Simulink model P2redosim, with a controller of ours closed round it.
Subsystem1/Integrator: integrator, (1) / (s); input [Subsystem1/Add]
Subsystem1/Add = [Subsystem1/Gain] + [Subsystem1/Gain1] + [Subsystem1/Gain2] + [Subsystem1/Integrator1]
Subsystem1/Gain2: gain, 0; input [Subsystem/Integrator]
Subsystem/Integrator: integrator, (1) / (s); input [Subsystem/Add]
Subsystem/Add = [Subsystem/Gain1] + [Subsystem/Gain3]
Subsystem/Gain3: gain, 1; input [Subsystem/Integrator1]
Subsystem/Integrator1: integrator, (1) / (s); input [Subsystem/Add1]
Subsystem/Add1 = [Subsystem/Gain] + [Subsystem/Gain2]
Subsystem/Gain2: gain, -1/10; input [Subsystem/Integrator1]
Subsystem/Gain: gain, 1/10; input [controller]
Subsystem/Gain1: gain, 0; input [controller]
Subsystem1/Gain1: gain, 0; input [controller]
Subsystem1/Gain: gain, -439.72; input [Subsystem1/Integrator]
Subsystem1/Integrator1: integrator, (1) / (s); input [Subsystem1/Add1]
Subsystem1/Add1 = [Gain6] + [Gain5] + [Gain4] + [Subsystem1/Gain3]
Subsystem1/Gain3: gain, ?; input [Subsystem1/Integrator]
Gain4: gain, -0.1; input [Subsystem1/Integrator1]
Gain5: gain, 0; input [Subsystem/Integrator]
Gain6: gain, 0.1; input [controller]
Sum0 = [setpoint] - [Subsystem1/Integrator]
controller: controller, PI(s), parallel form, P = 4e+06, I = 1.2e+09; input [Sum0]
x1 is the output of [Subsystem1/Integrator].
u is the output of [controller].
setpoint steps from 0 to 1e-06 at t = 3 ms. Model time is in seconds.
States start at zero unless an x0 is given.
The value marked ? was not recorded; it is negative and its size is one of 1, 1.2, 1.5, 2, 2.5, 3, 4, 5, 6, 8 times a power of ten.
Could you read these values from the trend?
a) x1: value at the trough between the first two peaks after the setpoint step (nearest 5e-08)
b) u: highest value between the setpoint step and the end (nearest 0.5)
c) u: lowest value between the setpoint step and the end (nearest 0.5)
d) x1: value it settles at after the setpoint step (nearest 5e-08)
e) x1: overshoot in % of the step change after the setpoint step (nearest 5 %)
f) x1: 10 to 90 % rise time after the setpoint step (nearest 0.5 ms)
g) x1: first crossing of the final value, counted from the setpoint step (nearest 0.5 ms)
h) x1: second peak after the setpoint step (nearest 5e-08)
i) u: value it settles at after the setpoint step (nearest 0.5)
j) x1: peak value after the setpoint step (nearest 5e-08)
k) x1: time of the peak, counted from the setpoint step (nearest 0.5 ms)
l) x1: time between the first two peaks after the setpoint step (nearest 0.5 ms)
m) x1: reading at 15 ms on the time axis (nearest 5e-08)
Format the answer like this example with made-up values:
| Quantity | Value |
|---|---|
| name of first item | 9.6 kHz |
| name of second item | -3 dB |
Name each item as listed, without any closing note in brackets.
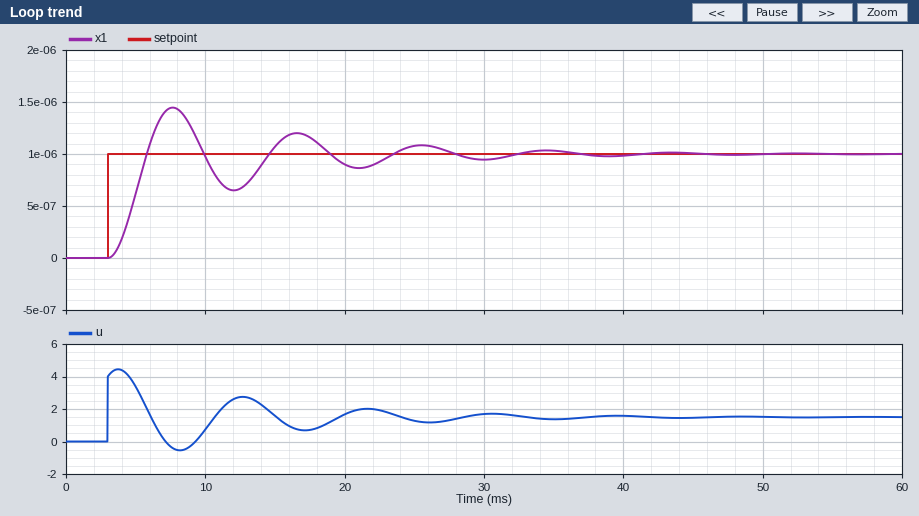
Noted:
| Quantity | Value |
|---|---|
| x1: value at the trough between the first two peaks after the setpoint step | 0.00000065 |
| u: highest value between the setpoint step and the end | 4.5 |
| u: lowest value between the setpoint step and the end | -0.5 |
| x1: value it settles at after the setpoint step | 0.00000100 |
| x1: overshoot in % of the step change after the setpoint step | 45 % |
| x1: 10 to 90 % rise time after the setpoint step | 2.0 ms |
| x1: first crossing of the final value, counted from the setpoint step | 3.0 ms |
| x1: second peak after the setpoint step | 0.00000120 |
| u: value it settles at after the setpoint step | 1.5 |
| x1: peak value after the setpoint step | 0.00000145 |
| x1: time of the peak, counted from the setpoint step | 4.5 ms |
| x1: time between the first two peaks after the setpoint step | 9.0 ms |
| x1: reading at 15 ms on the time axis | 0.00000105 |
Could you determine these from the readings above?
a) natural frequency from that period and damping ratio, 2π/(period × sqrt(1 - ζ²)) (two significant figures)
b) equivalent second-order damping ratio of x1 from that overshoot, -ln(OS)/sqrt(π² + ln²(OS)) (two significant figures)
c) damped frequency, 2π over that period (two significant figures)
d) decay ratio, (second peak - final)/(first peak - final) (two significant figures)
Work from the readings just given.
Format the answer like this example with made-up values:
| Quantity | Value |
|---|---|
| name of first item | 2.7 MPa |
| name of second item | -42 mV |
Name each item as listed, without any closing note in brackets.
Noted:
| Quantity | Value |
|---|---|
| natural frequency from that period and damping ratio, 2π/(period × sqrt(1 - ζ²)) | 0.72 rad/ms |
| equivalent second-order damping ratio of x1 from that overshoot, -ln(OS)/sqrt(π² + ln²(OS)) | 0.25 |
| damped frequency, 2π over that period | 0.70 rad/ms |
| decay ratio, (second peak - final)/(first peak - final) | 0.44 |
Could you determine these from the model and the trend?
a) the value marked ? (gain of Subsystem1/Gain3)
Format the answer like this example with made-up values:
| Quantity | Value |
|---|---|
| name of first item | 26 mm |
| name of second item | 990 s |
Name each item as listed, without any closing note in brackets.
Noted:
| Quantity | Value |
|---|---|
| the value marked ? | -150000 |
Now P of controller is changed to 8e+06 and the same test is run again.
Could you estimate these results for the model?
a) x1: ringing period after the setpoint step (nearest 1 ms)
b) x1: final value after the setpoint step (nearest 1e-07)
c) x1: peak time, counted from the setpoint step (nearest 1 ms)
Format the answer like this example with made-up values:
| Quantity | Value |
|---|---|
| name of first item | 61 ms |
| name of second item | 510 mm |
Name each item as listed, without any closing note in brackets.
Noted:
| Quantity | Value |
|---|---|
| x1: ringing period after the setpoint step | 7 ms |
| x1: final value after the setpoint step | 0.0000010 |
| x1: peak time, counted from the setpoint step | 3 ms |
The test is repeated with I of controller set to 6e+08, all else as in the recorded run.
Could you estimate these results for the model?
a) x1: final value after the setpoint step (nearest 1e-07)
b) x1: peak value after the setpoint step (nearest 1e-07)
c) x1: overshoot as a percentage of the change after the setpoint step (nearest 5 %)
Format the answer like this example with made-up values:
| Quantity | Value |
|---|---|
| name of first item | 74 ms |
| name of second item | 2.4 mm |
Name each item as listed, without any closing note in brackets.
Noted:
| Quantity | Value |
|---|---|
| x1: final value after the setpoint step | 0.0000010 |
| x1: peak value after the setpoint step | 0.0000012 |
| x1: overshoot as a percentage of the change after the setpoint step | 25 % |
